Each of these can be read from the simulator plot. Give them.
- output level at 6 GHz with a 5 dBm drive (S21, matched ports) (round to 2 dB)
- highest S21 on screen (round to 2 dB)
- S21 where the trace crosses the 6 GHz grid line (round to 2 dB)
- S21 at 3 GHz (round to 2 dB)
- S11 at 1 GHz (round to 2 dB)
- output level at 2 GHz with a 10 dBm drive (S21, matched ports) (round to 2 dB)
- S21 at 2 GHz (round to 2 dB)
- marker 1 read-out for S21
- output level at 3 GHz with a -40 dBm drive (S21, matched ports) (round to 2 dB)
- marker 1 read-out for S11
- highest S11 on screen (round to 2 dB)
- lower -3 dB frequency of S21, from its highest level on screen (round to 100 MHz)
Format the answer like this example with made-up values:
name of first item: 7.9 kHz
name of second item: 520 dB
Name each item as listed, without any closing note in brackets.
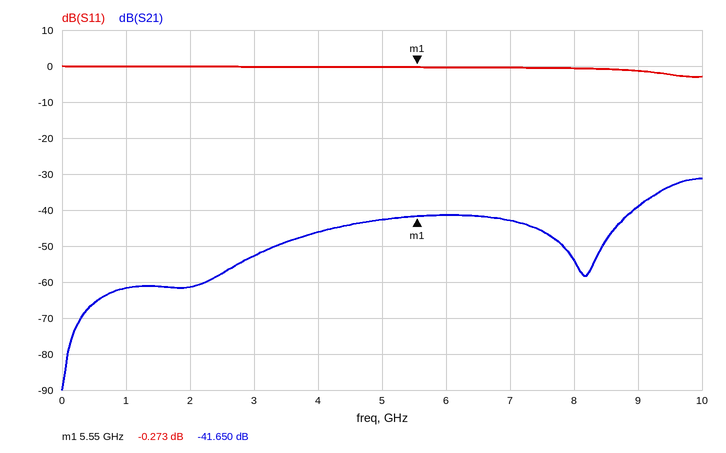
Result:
output level at 6 GHz with a 5 dBm drive (S21, matched ports): -36 dBm
highest S21 on screen: -32 dB
S21 where the trace crosses the 6 GHz grid line: -42 dB
S21 at 3 GHz: -52 dB
S11 at 1 GHz: 0 dB
output level at 2 GHz with a 10 dBm drive (S21, matched ports): -52 dBm
S21 at 2 GHz: -62 dB
marker 1 read-out for S21: -41.650 dB
output level at 3 GHz with a -40 dBm drive (S21, matched ports): -92 dBm
marker 1 read-out for S11: -0.273 dB
highest S11 on screen: 0 dB
lower -3 dB frequency of S21, from its highest level on screen: 9.4 GHz
